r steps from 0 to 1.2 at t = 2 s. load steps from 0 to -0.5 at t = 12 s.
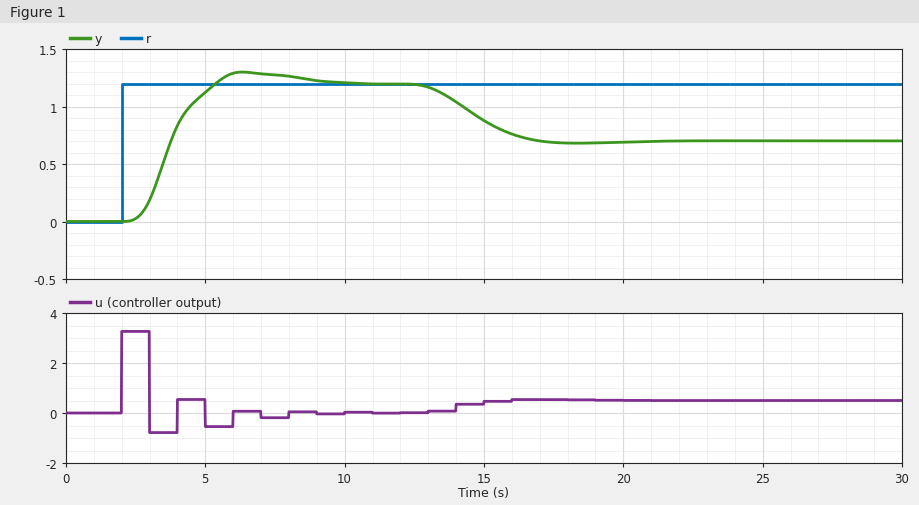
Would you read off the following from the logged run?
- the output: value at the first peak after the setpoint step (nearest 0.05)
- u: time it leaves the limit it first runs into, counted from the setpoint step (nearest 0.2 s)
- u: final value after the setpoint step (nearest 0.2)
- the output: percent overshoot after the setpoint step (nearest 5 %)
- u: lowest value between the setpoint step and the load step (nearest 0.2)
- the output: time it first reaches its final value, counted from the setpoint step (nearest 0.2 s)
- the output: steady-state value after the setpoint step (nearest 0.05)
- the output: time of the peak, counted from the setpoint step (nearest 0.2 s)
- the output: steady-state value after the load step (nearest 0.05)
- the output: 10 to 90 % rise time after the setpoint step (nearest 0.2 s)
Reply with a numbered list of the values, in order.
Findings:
1. 1.30
2. 1.0 s
3. 0.0
4. 10 %
5. -0.8
6. 3.4 s
7. 1.20
8. 4.4 s
9. 0.70
10. 2.0 s
